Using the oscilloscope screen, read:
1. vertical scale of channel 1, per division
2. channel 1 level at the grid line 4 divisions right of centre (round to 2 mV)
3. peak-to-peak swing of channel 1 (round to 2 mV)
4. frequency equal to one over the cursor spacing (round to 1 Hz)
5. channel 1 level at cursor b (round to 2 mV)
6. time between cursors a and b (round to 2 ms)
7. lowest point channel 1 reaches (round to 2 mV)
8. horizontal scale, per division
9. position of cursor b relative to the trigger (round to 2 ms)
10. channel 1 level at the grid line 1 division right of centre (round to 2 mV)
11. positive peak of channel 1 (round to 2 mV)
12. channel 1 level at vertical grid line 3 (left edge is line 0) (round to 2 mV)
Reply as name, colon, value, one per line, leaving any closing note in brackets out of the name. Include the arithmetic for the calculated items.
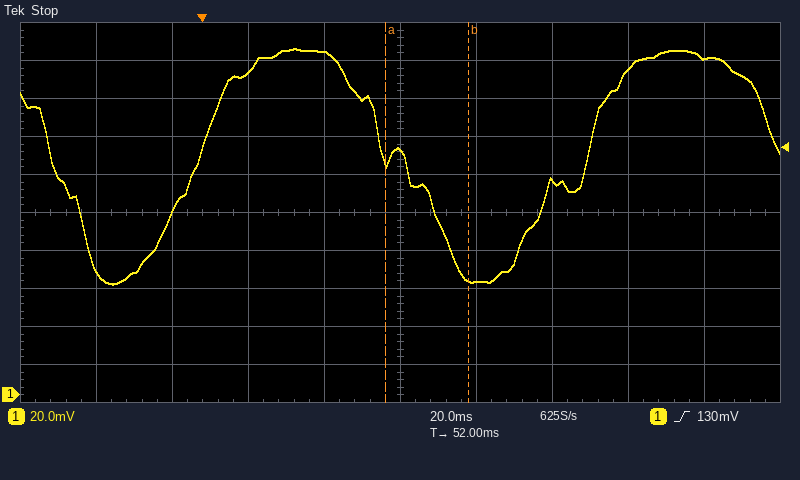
vertical scale of channel 1, per division: 20 mV
channel 1 level at the grid line 4 divisions right of centre: 178 mV
peak-to-peak swing of channel 1: 182 mV − (58 mV) = 124 mV
frequency equal to one over the cursor spacing: 1 / 22 ms ≈ 45 Hz
channel 1 level at cursor b: 60 mV
time between cursors a and b: 22 ms
lowest point channel 1 reaches: 58 mV
horizontal scale, per division: 20 ms
position of cursor b relative to the trigger: +70 ms
channel 1 level at the grid line 1 division right of centre: 60 mV
positive peak of channel 1: 182 mV
channel 1 level at vertical grid line 3 (left edge is line 0): 170 mV
